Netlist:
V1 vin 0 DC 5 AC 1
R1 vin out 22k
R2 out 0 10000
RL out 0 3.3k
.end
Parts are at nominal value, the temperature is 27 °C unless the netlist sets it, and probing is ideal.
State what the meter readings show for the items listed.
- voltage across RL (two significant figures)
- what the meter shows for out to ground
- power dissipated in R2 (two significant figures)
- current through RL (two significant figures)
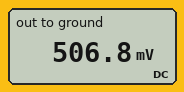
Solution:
510 mV
506.8 mV
26 µW
150 µA
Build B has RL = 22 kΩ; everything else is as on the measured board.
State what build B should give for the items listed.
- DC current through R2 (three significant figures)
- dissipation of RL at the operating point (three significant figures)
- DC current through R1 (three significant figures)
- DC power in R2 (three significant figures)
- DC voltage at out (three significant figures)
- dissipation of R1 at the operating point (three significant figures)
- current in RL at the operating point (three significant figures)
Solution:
119 µA
64.4 µW
173 µA
142 µW
1.19 V
660 µW
54.1 µA
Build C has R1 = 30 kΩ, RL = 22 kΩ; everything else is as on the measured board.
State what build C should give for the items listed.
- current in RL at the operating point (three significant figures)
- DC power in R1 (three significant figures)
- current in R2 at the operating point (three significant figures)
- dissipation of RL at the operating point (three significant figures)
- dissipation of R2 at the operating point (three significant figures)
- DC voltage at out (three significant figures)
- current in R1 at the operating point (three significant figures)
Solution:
42.4 µA
552 µW
93.2 µA
39.5 µW
86.9 µW
932 mV
136 µA
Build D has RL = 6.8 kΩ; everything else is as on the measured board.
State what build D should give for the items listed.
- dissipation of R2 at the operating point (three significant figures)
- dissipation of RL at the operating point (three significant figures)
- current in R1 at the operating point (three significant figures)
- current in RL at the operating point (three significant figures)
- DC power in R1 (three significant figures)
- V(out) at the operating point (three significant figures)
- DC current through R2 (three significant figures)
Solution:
60.4 µW
88.8 µW
192 µA
114 µA
811 µW
777 mV
77.7 µA
